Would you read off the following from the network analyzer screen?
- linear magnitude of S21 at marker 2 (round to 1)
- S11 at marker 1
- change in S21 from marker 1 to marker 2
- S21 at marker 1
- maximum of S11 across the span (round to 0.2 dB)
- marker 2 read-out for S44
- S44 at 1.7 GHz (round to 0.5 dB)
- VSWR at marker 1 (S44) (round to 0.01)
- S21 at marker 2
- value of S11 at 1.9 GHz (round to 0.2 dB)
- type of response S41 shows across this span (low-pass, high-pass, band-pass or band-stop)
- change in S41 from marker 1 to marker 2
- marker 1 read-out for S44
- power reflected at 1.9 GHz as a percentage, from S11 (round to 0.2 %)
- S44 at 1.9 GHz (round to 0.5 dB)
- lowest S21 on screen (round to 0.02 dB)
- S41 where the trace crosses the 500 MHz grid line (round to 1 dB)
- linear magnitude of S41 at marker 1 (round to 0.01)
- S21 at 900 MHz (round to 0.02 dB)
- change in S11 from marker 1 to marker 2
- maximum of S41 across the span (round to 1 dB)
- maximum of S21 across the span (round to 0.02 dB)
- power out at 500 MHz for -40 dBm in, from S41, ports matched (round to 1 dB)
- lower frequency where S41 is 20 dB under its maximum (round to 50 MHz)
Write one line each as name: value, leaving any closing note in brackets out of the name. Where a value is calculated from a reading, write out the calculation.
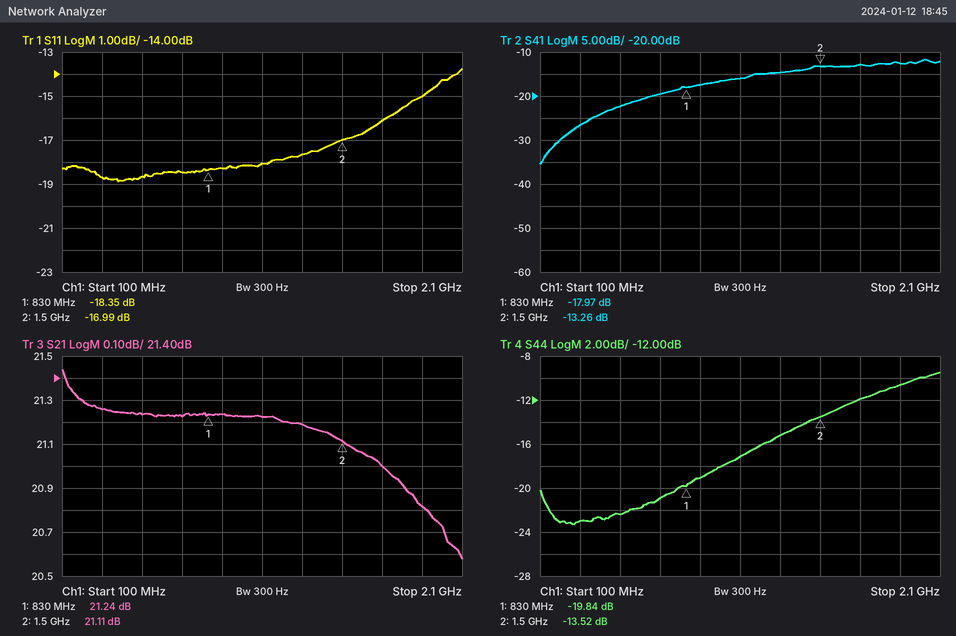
linear magnitude of S21 at marker 2: 10^(21.11/20) ≈ 11
S11 at marker 1: -18.35 dB
change in S21 from marker 1 to marker 2: 21.11 − (21.24) = -0.13 dB
S21 at marker 1: 21.24 dB
maximum of S11 across the span: -13.8 dB
marker 2 read-out for S44: -13.52 dB
S44 at 1.7 GHz: -12.0 dB
VSWR at marker 1 (S44): (1 + 0.1019)/(1 − 0.1019) ≈ 1.23
S21 at marker 2: 21.11 dB
value of S11 at 1.9 GHz: -15.0 dB
type of response S41 shows across this span: high-pass
change in S41 from marker 1 to marker 2: -13.26 − (-17.97) = 4.71 dB
marker 1 read-out for S44: -19.84 dB
power reflected at 1.9 GHz as a percentage, from S11: 10^(-15/10) ≈ 3.2 %
S44 at 1.9 GHz: -10.5 dB
lowest S21 on screen: 20.58 dB
S41 where the trace crosses the 500 MHz grid line: -22 dB
linear magnitude of S41 at marker 1: 10^(-17.97/20) ≈ 0.13
S21 at 900 MHz: 21.24 dB
change in S11 from marker 1 to marker 2: -16.99 − (-18.35) = 1.36 dB
maximum of S41 across the span: -12 dB
maximum of S21 across the span: 21.44 dB
power out at 500 MHz for -40 dBm in, from S41, ports matched: -40 dBm + (-22 dB) = -62 dBm
lower frequency where S41 is 20 dB under its maximum: 150 MHz
